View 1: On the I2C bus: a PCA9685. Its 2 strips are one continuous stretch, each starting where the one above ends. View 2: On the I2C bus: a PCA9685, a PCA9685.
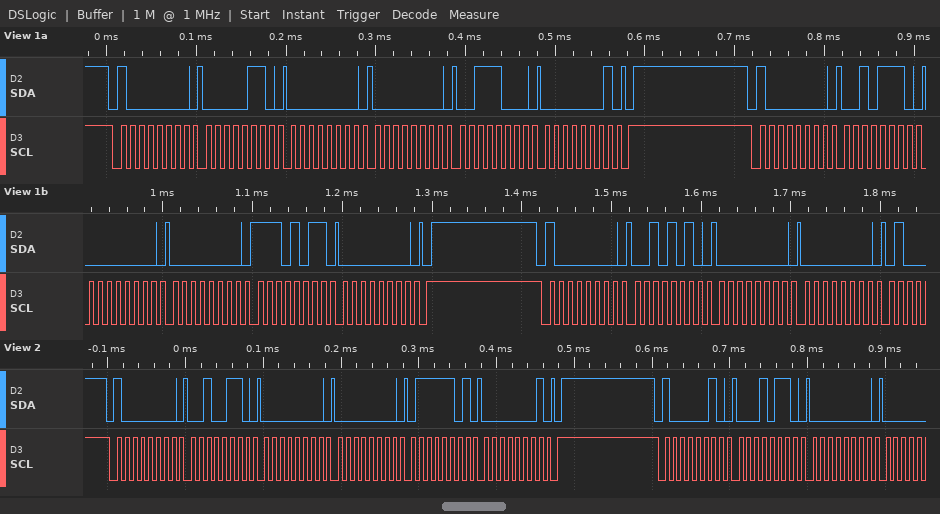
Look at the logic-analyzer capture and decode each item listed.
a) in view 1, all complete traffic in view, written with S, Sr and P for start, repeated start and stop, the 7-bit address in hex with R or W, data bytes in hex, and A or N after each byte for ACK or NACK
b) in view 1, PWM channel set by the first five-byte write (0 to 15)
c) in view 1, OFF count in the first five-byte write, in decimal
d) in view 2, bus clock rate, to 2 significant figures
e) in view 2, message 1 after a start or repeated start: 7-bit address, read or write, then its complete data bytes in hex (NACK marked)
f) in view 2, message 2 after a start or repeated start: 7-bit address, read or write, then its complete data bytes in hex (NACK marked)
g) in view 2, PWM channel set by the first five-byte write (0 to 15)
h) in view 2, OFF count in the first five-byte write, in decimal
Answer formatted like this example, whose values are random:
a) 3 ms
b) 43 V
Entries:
a) S 40W A 06 A 00 A 00 A 38 A 01 A P S 40W A 2E A 00 A 00 A EB A 00 A P S 40W A 2A A 00 A 00 A
b) 0
c) 312
d) 100 kHz
e) 0x40 write: 26 00 00 7D 01
f) 0x41 write: 16 00
g) 8
h) 381
